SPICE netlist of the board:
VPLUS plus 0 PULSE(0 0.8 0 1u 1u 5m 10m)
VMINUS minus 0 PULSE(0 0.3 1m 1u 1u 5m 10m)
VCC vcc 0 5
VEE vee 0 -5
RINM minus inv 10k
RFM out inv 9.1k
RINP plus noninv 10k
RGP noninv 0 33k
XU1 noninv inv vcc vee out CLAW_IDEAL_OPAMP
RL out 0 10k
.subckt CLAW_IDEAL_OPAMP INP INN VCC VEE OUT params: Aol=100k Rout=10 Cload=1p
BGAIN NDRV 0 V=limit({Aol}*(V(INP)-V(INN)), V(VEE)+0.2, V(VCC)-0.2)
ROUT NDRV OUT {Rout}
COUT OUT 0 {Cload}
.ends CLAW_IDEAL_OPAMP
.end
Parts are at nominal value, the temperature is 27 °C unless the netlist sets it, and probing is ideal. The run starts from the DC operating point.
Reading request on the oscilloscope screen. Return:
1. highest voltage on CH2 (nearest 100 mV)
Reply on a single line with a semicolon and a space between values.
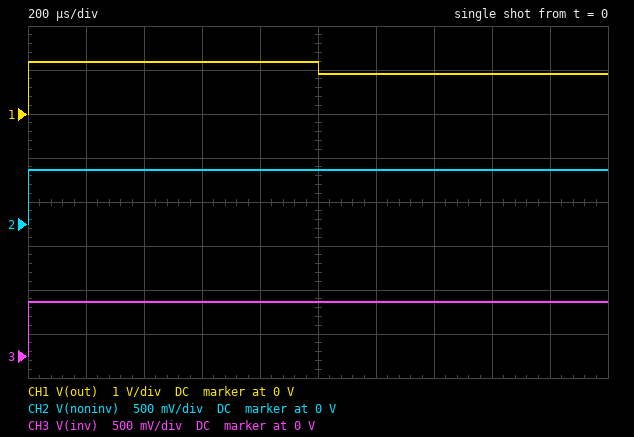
600 mV
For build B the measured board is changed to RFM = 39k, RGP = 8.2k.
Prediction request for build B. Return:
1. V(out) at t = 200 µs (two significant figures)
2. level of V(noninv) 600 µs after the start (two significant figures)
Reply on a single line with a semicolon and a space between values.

1.8 V; 360 mV
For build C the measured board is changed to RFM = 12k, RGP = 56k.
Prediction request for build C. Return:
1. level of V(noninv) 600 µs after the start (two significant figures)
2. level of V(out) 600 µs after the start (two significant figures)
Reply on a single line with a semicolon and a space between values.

680 mV; 1.5 V
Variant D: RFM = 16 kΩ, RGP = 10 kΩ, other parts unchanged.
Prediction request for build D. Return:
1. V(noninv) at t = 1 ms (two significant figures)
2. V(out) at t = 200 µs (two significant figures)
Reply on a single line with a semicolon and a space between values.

400 mV; 1.0 V
